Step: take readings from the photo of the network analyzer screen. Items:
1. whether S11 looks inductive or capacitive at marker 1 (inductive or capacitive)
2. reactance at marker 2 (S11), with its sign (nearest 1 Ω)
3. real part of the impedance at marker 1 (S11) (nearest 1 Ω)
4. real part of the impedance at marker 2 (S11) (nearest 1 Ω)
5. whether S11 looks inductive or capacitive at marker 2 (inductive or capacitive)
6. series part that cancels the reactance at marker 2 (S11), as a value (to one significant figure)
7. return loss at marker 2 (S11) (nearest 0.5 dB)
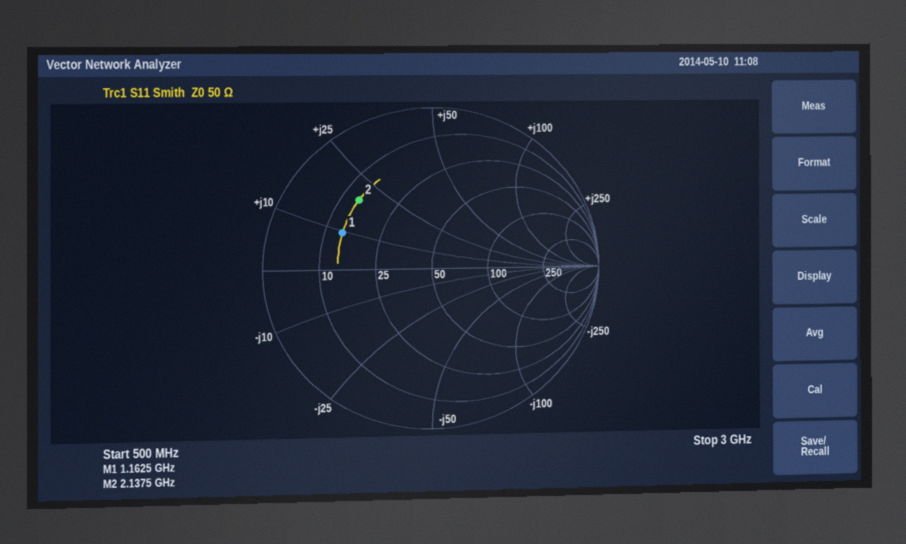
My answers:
inductive
+19 Ω
14 Ω
14 Ω
inductive
4 pF
4.5 dB
